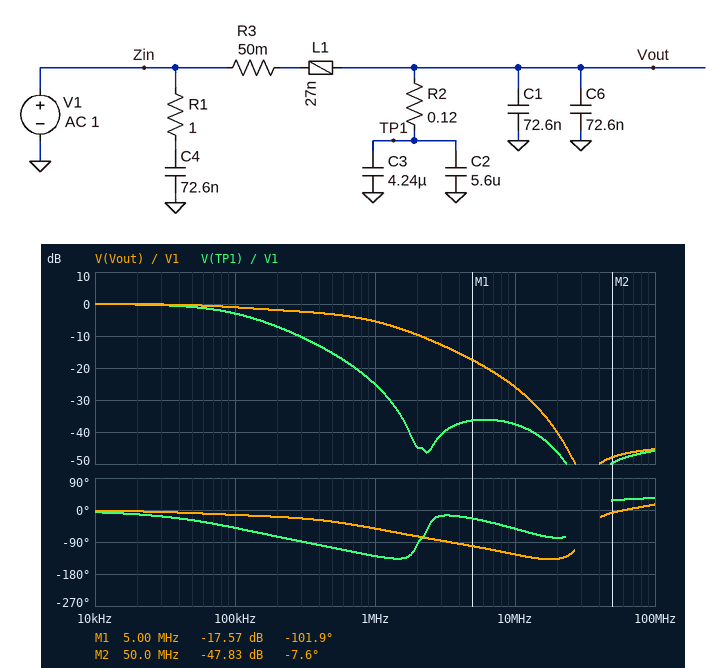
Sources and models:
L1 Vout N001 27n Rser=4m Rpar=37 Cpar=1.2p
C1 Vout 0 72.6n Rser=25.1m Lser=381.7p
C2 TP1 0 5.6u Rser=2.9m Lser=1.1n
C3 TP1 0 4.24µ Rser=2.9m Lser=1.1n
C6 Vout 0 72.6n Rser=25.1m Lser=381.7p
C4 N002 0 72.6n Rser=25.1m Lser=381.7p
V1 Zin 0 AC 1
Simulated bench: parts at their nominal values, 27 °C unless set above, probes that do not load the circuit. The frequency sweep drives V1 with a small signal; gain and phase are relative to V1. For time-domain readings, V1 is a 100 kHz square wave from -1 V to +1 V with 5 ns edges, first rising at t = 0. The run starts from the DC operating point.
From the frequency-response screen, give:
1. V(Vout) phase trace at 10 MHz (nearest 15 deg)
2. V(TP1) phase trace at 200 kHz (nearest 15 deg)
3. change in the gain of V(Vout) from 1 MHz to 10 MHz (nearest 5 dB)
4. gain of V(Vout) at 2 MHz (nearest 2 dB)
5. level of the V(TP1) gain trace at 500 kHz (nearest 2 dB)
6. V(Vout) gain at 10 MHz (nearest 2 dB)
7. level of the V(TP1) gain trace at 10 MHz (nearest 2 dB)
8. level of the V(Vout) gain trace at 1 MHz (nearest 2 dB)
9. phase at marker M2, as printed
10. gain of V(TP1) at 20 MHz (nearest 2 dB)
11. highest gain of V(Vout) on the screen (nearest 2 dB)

-120 deg
-75 deg
-20 dB
-10 dB
-16 dB
-26 dB
-38 dB
-6 dB
-7.6 deg
-46 dB
0 dB
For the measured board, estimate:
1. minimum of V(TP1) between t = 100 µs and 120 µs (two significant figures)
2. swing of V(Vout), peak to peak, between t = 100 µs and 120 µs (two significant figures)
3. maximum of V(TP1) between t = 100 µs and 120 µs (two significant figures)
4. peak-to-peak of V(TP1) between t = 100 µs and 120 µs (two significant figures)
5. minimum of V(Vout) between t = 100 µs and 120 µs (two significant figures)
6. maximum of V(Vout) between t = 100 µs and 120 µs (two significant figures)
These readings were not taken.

-910 mV
2.0 V
910 mV
1.8 V
-980 mV
980 mV
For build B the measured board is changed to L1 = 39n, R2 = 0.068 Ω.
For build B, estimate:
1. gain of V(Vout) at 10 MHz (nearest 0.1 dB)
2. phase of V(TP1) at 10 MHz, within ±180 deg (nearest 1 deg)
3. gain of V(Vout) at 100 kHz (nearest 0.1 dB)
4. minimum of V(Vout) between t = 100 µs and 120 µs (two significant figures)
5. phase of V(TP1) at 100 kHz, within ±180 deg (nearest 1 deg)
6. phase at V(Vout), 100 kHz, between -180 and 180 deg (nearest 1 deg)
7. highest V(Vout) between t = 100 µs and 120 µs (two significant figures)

-30.5 dB
-40 deg
-0.4 dB
-1.0 V
-42 deg
-19 deg
1.0 V
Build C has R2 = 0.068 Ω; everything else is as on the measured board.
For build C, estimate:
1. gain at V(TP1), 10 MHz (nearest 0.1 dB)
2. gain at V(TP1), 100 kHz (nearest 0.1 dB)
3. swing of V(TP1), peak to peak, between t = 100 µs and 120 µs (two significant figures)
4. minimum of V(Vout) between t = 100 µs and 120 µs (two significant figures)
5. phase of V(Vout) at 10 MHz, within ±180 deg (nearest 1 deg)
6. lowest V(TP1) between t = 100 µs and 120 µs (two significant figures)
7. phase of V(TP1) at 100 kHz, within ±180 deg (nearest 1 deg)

-34.7 dB
-1.4 dB
2.0 V
-1.0 V
-102 deg
-990 mV
-40 deg
